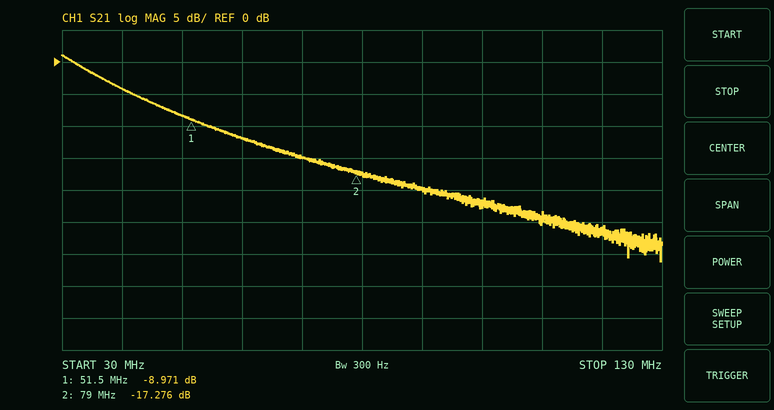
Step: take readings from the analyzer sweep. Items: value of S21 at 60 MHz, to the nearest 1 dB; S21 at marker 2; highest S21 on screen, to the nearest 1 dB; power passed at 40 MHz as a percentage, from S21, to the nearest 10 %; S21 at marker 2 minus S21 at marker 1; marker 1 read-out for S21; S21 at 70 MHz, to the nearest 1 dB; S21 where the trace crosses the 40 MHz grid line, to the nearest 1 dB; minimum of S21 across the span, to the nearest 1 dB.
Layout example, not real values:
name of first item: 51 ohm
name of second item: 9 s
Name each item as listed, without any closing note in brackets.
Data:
value of S21 at 60 MHz, to the nearest 1 dB: -12 dB
S21 at marker 2: -17.276 dB
highest S21 on screen, to the nearest 1 dB: 1 dB
power passed at 40 MHz as a percentage, from S21, to the nearest 10 %: 40 %
S21 at marker 2 minus S21 at marker 1: -8.305 dB
marker 1 read-out for S21: -8.971 dB
S21 at 70 MHz, to the nearest 1 dB: -15 dB
S21 where the trace crosses the 40 MHz grid line, to the nearest 1 dB: -4 dB
minimum of S21 across the span, to the nearest 1 dB: -31 dB
